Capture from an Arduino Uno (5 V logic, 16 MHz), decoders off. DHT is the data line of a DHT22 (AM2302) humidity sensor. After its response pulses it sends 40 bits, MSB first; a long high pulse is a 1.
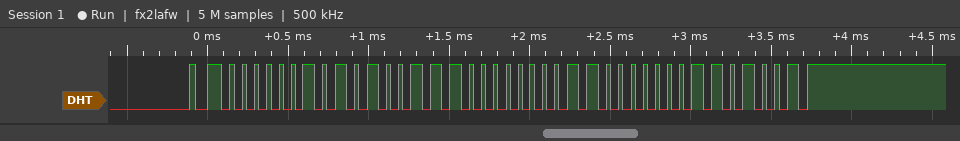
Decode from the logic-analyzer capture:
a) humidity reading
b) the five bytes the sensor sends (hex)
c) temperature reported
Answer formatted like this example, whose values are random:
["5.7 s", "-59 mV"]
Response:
["67.9 %", "02 A7 00 C0 69", "19.2 °C"]
